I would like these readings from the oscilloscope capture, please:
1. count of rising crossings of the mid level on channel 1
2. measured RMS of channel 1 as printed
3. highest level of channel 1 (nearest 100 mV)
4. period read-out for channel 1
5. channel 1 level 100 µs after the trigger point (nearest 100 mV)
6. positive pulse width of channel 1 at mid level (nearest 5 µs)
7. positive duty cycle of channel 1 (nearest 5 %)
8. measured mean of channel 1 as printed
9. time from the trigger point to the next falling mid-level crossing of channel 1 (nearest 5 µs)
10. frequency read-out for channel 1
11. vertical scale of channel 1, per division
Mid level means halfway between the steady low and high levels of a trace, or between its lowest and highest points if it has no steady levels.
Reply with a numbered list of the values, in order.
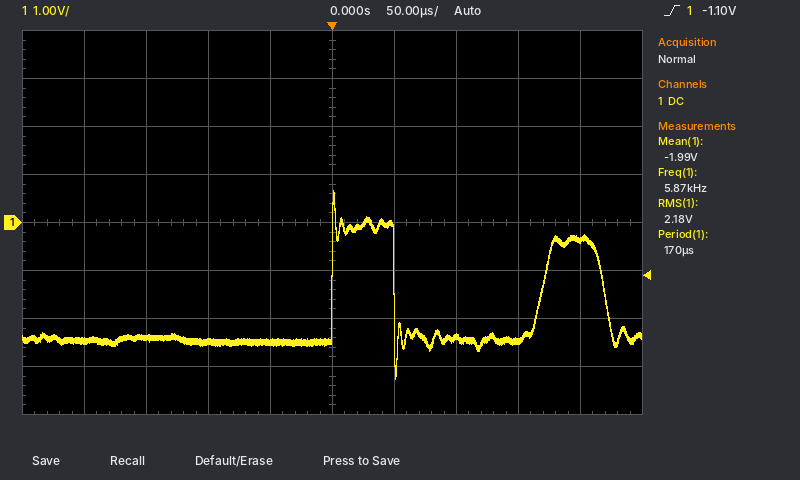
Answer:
1. 2
2. 2.18 V
3. 700 mV
4. 170 µs
5. -2.4 V
6. 50 µs
7. 30 %
8. -1.99 V
9. 50 µs
10. 5.87 kHz
11. 1 V
